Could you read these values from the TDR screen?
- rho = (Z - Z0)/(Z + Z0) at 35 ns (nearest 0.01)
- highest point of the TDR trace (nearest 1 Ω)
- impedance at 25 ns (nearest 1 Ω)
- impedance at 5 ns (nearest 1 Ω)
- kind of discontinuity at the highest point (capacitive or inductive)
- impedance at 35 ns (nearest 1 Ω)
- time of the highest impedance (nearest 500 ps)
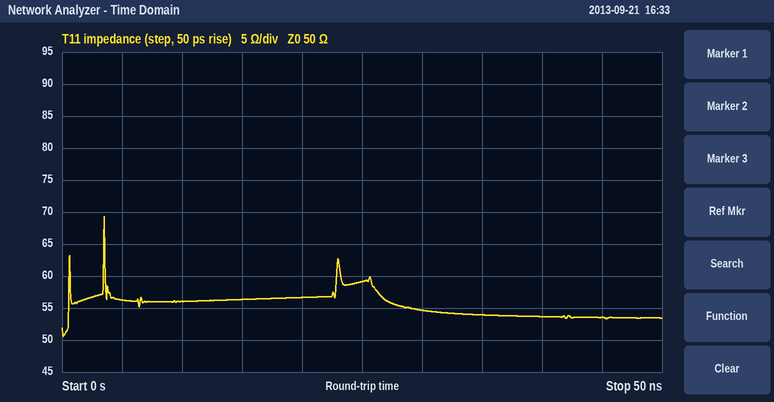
+0.04
69 Ω
59 Ω
56 Ω
inductive
54 Ω
3.5 ns
